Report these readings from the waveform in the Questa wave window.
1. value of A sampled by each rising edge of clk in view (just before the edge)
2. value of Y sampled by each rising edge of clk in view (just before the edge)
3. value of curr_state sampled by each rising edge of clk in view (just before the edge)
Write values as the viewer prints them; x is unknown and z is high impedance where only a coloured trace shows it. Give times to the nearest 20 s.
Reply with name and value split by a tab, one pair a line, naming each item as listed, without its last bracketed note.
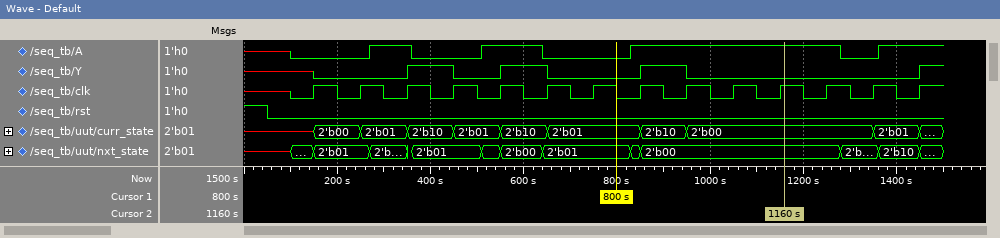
value of A sampled by each rising edge of clk in view	0 0 1 0 1 0 0 1 1 1 1 1 0 1
value of Y sampled by each rising edge of clk in view	x 0 0 1 0 1 0 0 1 0 0 0 0 0
value of curr_state sampled by each rising edge of clk in view	x, 2'b00, 2'b01, 2'b10, 2'b01, 2'b10, 2'b01, 2'b01, 2'b10, 2'b00, 2'b00, 2'b00, 2'b00, 2'b01
